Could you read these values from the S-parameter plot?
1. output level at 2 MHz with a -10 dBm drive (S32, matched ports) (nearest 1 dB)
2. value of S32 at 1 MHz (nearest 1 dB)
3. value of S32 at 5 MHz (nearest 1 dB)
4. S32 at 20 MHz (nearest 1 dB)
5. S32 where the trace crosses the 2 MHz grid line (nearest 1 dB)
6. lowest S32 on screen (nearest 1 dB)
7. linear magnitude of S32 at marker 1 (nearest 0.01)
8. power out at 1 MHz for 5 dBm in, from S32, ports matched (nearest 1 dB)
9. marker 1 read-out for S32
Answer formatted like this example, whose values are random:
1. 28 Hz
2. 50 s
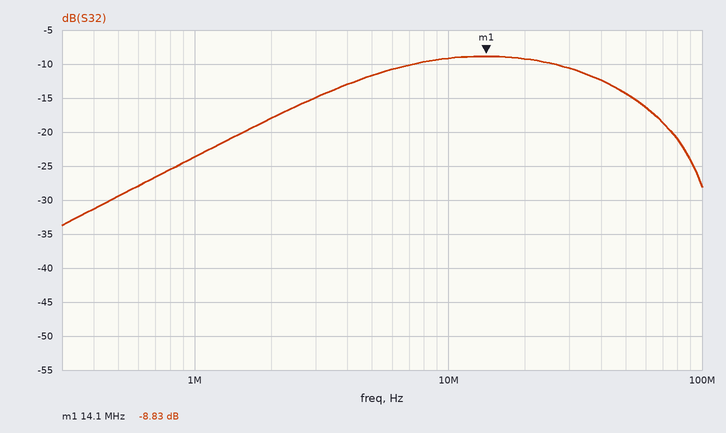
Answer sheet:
1. -28 dBm
2. -24 dB
3. -12 dB
4. -9 dB
5. -18 dB
6. -34 dB
7. 0.36
8. -19 dBm
9. -8.83 dB
